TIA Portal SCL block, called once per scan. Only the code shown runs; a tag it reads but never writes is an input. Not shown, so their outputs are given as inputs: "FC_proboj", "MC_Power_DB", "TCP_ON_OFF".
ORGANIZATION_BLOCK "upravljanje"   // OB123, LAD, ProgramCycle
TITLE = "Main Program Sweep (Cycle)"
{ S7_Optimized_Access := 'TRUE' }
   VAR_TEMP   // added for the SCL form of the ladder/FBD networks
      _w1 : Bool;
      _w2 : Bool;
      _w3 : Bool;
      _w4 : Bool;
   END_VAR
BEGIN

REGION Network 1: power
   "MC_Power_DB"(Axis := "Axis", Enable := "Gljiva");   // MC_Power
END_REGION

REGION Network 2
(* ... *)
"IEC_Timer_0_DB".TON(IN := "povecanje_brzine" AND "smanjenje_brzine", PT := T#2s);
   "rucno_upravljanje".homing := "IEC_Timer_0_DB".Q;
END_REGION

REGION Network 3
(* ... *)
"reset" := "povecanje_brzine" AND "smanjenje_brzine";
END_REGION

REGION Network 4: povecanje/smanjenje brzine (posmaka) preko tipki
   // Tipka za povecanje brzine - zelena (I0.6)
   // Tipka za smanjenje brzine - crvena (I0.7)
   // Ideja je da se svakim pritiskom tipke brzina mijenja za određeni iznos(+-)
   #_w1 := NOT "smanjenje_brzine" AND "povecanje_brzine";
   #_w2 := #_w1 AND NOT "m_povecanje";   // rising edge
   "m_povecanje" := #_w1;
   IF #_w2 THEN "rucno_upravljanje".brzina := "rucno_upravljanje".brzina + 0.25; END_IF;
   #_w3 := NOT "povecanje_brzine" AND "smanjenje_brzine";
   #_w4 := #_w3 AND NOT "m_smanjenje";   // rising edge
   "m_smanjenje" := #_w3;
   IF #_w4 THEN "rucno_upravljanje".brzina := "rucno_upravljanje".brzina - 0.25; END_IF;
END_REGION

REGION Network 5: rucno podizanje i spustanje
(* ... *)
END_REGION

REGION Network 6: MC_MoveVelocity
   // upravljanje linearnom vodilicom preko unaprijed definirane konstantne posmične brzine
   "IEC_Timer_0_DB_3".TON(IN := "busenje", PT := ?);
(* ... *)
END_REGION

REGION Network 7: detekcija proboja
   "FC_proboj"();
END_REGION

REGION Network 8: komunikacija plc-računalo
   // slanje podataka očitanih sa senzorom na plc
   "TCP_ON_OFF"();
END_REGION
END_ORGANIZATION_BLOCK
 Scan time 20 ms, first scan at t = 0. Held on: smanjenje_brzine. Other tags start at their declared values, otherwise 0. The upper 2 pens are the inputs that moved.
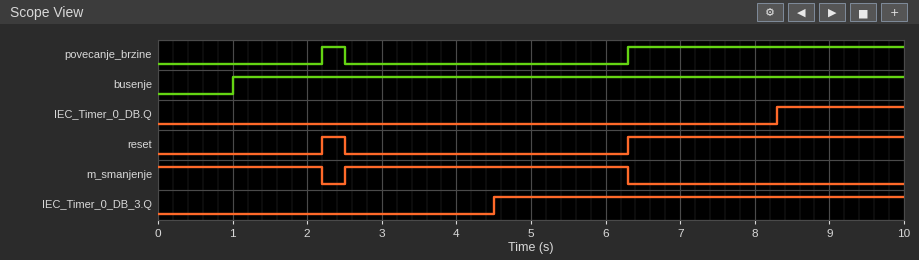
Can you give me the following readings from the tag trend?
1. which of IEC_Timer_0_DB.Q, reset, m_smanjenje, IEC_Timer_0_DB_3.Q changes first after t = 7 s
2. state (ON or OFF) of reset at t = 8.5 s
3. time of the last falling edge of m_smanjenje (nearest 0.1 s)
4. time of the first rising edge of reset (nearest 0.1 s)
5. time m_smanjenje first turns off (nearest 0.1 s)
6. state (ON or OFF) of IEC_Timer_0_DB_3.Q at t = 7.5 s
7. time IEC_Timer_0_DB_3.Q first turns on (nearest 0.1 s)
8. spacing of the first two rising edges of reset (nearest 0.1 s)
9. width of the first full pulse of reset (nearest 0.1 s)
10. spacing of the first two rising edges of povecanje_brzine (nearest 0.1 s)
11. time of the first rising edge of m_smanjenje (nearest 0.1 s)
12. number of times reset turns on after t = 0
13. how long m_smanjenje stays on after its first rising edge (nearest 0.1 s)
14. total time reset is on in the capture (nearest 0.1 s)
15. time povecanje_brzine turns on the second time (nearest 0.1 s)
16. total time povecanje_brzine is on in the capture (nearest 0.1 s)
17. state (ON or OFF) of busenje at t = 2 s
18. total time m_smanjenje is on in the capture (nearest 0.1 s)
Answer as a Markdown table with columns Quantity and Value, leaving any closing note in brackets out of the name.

| Quantity | Value |
|---|---|
| which of IEC_Timer_0_DB.Q, reset, m_smanjenje, IEC_Timer_0_DB_3.Q changes first after t = 7 s | IEC_Timer_0_DB.Q |
| state (ON or OFF) of reset at t = 8.5 s | ON |
| time of the last falling edge of m_smanjenje | 6.3 s |
| time of the first rising edge of reset | 2.2 s |
| time m_smanjenje first turns off | 2.2 s |
| state (ON or OFF) of IEC_Timer_0_DB_3.Q at t = 7.5 s | ON |
| time IEC_Timer_0_DB_3.Q first turns on | 4.5 s |
| spacing of the first two rising edges of reset | 4.1 s |
| width of the first full pulse of reset | 0.3 s |
| spacing of the first two rising edges of povecanje_brzine | 4.1 s |
| time of the first rising edge of m_smanjenje | 2.5 s |
| number of times reset turns on after t = 0 | 2 |
| how long m_smanjenje stays on after its first rising edge | 3.8 s |
| total time reset is on in the capture | 4.0 s |
| time povecanje_brzine turns on the second time | 6.3 s |
| total time povecanje_brzine is on in the capture | 4.0 s |
| state (ON or OFF) of busenje at t = 2 s | ON |
| total time m_smanjenje is on in the capture | 6.0 s |
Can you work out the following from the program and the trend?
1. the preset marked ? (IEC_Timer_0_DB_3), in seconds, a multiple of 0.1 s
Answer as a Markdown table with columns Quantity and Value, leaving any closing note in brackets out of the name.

| Quantity | Value |
|---|---|
| the preset marked ? (IEC_Timer_0_DB_3), in seconds, a multiple of 0.1 s | 3.5 s |
